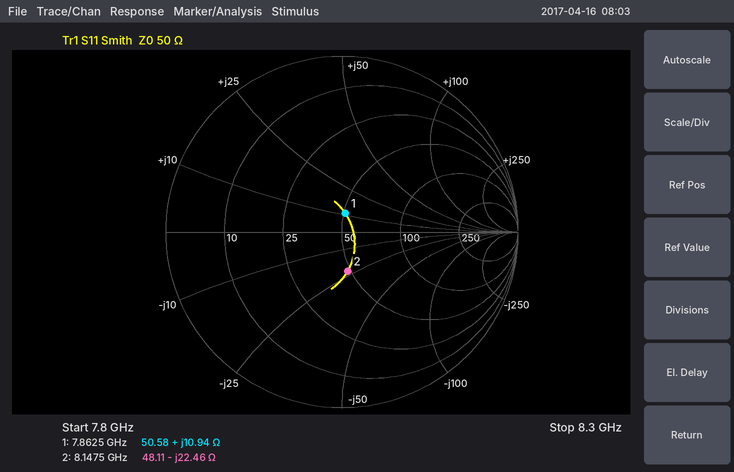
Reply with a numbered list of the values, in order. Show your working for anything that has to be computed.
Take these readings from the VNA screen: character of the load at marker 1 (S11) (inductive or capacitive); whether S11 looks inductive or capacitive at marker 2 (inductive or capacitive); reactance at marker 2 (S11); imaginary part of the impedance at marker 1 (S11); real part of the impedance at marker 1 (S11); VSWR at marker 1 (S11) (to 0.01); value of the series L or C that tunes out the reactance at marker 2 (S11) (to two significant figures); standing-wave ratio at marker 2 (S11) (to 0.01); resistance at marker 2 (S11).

1. inductive
2. capacitive
3. -22.46 Ω
4. +10.94 Ω
5. 50.58 Ω
6. 1.24
7. L = 22.46 Ω/(2π × 8.1475 GHz) ≈ 439 pH, so 440 pH to two significant figures
8. 1.58
9. 48.11 Ω
